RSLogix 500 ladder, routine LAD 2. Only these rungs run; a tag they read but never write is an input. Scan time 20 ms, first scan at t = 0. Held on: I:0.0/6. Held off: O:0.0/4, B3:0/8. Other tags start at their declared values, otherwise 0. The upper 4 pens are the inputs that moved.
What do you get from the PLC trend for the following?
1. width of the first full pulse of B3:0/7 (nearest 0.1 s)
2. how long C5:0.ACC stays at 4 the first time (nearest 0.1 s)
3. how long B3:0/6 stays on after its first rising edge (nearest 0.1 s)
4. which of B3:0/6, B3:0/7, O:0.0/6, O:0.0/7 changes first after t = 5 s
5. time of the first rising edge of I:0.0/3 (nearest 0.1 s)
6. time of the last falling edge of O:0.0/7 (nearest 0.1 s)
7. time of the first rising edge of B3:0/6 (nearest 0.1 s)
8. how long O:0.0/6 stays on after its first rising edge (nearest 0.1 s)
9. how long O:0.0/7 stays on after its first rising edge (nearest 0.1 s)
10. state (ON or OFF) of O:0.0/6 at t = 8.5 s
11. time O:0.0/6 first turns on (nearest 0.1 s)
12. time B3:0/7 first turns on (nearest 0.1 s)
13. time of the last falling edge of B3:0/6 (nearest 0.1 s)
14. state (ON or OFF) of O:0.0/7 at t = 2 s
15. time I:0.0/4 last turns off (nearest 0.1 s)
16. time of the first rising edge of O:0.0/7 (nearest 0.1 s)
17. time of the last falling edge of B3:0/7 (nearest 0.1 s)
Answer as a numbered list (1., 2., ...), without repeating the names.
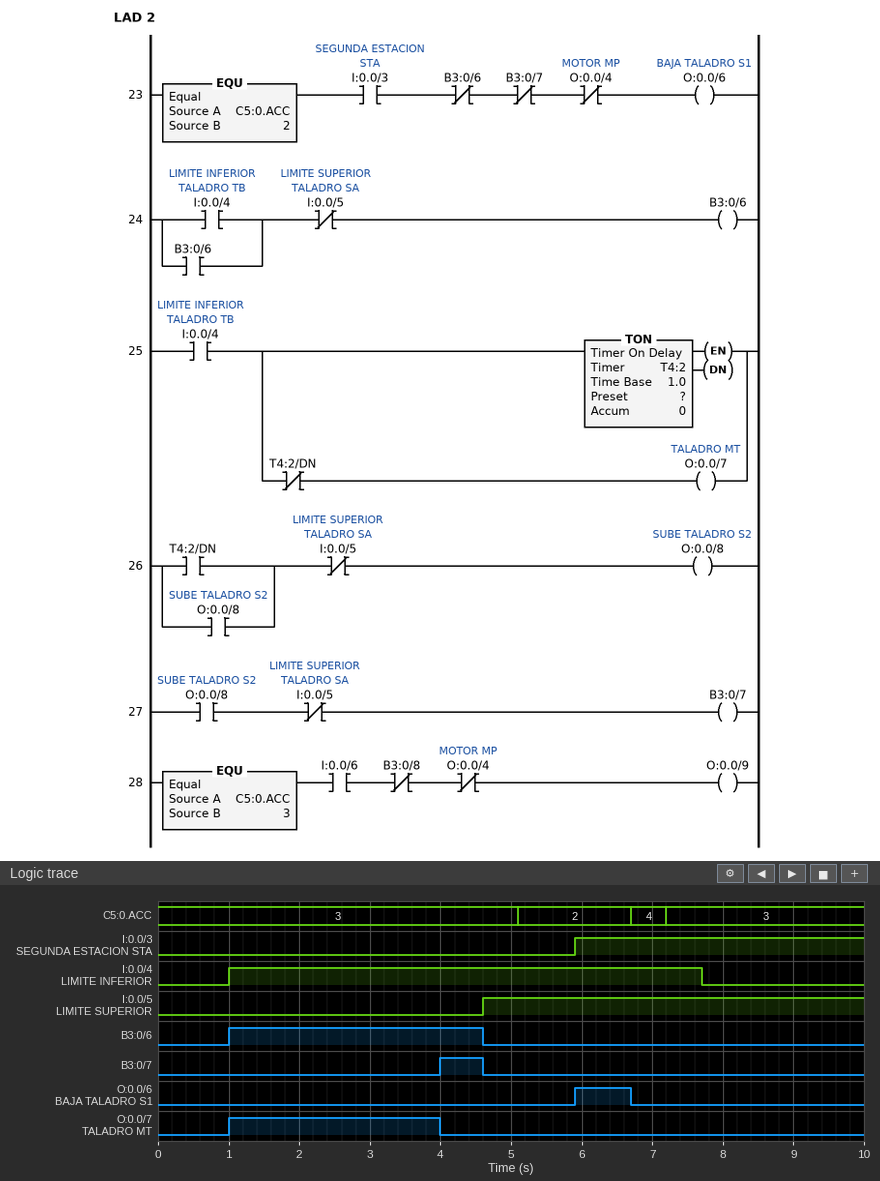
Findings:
1. 0.6 s
2. 0.5 s
3. 3.6 s
4. O:0.0/6
5. 5.9 s
6. 4.0 s
7. 1.0 s
8. 0.8 s
9. 3.0 s
10. OFF
11. 5.9 s
12. 4.0 s
13. 4.6 s
14. ON
15. 7.7 s
16. 1.0 s
17. 4.6 s
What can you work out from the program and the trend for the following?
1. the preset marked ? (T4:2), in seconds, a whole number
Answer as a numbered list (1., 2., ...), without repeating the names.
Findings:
1. 3 s
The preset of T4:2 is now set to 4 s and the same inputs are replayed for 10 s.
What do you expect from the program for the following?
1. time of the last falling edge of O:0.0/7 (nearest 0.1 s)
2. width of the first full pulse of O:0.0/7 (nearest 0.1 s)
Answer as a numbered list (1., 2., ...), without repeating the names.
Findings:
1. 5.0 s
2. 4.0 s
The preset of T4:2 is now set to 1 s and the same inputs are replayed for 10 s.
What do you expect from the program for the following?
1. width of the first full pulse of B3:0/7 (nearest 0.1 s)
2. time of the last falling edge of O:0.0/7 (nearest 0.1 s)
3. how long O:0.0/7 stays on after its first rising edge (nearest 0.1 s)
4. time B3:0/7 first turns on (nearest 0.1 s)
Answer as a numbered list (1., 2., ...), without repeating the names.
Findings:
1. 2.6 s
2. 2.0 s
3. 1.0 s
4. 2.0 s
